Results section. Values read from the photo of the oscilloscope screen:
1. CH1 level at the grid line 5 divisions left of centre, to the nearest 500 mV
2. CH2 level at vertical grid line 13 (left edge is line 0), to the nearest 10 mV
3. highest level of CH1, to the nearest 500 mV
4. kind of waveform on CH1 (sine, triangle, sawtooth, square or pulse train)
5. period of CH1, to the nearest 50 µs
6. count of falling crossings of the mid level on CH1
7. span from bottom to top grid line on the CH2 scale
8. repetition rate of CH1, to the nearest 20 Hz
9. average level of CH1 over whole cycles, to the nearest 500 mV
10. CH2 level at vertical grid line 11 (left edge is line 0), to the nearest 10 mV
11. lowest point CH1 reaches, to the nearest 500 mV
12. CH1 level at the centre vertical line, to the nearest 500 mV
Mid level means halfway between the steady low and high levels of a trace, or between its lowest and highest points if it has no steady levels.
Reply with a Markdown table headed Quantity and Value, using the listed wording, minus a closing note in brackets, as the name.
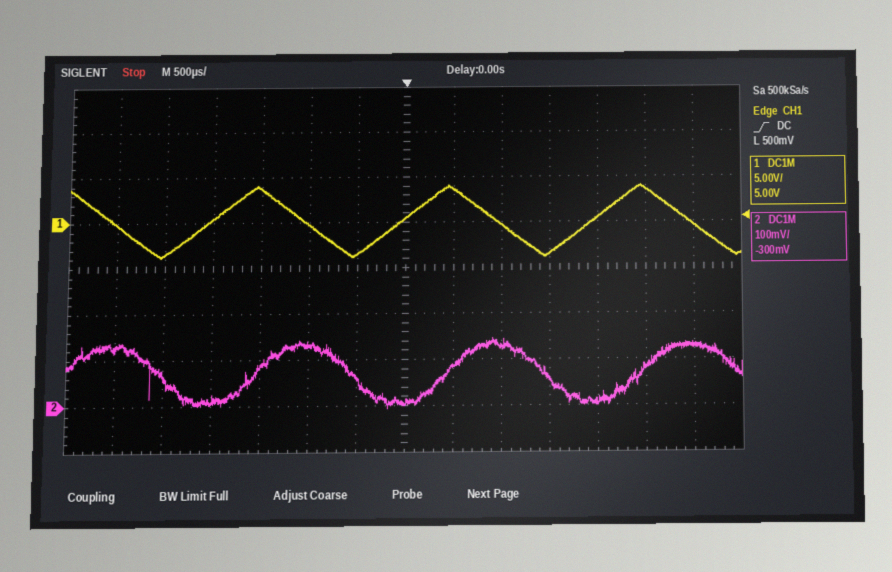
| Quantity | Value |
|---|---|
| CH1 level at the grid line 5 divisions left of centre, to the nearest 500 mV | -3.5 V |
| CH2 level at vertical grid line 13 (left edge is line 0), to the nearest 10 mV | 130 mV |
| highest level of CH1, to the nearest 500 mV | 4.0 V |
| kind of waveform on CH1 | triangle |
| period of CH1, to the nearest 50 µs | 2.00 ms |
| count of falling crossings of the mid level on CH1 | 4 |
| span from bottom to top grid line on the CH2 scale | 800 mV |
| repetition rate of CH1, to the nearest 20 Hz | 500 Hz |
| average level of CH1 over whole cycles, to the nearest 500 mV | 0.0 V |
| CH2 level at vertical grid line 11 (left edge is line 0), to the nearest 10 mV | 10 mV |
| lowest point CH1 reaches, to the nearest 500 mV | -4.0 V |
| CH1 level at the centre vertical line, to the nearest 500 mV | 500 mV |
